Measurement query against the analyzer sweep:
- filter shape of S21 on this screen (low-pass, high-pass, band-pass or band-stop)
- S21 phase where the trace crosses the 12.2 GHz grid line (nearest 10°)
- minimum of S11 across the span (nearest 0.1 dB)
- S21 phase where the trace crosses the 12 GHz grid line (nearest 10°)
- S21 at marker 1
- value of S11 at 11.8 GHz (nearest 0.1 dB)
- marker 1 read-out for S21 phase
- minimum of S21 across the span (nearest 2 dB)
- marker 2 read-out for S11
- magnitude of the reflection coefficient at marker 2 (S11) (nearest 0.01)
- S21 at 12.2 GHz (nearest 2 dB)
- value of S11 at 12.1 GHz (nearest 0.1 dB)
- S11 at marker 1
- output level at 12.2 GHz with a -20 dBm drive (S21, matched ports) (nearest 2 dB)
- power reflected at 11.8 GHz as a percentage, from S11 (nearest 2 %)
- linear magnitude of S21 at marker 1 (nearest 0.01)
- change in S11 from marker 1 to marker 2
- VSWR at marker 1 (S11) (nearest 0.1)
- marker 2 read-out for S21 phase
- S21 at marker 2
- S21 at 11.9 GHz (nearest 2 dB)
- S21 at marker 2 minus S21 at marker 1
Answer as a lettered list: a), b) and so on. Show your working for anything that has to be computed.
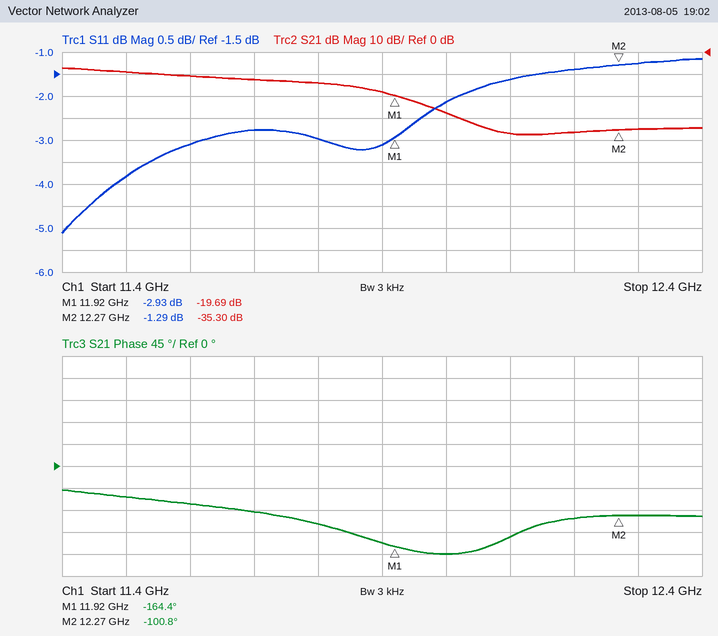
a) low-pass
b) -110°
c) -5.1 dB
d) -180°
e) -19.69 dB
f) -3.0 dB
g) -164.4°
h) -38 dB
i) -1.29 dB
j) 10^(-1.29/20) ≈ 0.86
k) -36 dB
l) -1.6 dB
m) -2.93 dB
n) -20 dBm + (-36 dB) = -56 dBm
o) 10^(-3/10) ≈ 50 %
p) 10^(-19.69/20) ≈ 0.10
q) -1.29 − (-2.93) = 1.64 dB
r) (1 + 0.7137)/(1 − 0.7137) ≈ 6.0
s) -100.8°
t) -35.30 dB
u) -18 dB
v) -35.3 − (-19.69) = -15.61 dB
